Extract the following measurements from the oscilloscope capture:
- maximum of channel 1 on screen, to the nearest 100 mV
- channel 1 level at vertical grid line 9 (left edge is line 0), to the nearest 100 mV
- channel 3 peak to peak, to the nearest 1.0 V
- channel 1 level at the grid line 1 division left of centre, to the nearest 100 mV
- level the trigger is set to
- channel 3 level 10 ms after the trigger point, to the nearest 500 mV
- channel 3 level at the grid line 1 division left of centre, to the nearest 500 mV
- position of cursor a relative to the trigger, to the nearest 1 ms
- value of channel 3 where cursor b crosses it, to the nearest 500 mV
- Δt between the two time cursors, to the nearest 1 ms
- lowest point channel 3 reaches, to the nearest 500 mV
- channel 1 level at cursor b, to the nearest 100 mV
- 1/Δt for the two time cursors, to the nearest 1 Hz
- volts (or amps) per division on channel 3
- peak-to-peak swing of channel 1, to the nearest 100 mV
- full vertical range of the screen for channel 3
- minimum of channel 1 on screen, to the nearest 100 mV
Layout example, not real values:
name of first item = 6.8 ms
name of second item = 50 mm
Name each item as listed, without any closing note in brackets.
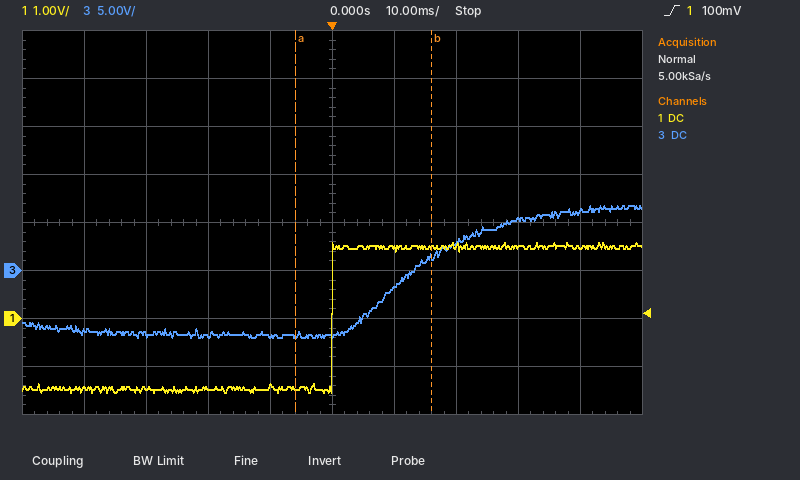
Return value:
maximum of channel 1 on screen, to the nearest 100 mV = 1.6 V
channel 1 level at vertical grid line 9 (left edge is line 0), to the nearest 100 mV = 1.5 V
channel 3 peak to peak, to the nearest 1.0 V = 14.0 V
channel 1 level at the grid line 1 division left of centre, to the nearest 100 mV = -1.4 V
level the trigger is set to = 100 mV
channel 3 level 10 ms after the trigger point, to the nearest 500 mV = -1.5 V
channel 3 level at the grid line 1 division left of centre, to the nearest 500 mV = -7.0 V
position of cursor a relative to the trigger, to the nearest 1 ms = -6 ms
value of channel 3 where cursor b crosses it, to the nearest 500 mV = 1.5 V
Δt between the two time cursors, to the nearest 1 ms = 22 ms
lowest point channel 3 reaches, to the nearest 500 mV = -7.0 V
channel 1 level at cursor b, to the nearest 100 mV = 1.5 V
1/Δt for the two time cursors, to the nearest 1 Hz = 45 Hz
volts (or amps) per division on channel 3 = 5 V
peak-to-peak swing of channel 1, to the nearest 100 mV = 3.1 V
full vertical range of the screen for channel 3 = 40 V
minimum of channel 1 on screen, to the nearest 100 mV = -1.5 V
